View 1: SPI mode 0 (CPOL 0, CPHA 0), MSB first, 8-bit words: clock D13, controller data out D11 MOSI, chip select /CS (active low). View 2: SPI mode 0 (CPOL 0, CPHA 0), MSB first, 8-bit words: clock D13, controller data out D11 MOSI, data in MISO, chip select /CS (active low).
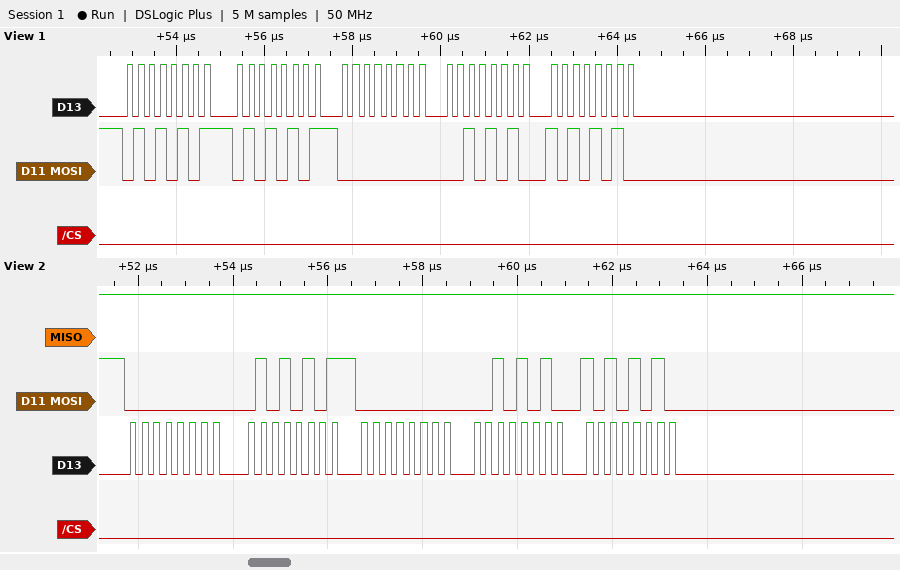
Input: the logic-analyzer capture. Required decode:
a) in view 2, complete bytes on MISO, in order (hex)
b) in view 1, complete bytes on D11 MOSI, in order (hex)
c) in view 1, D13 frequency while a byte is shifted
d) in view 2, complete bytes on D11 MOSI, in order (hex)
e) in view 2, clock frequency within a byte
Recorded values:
FF FF FF FF FF
55 55 00 2A AA
4 MHz
00 55 00 2A AA
4 MHz
